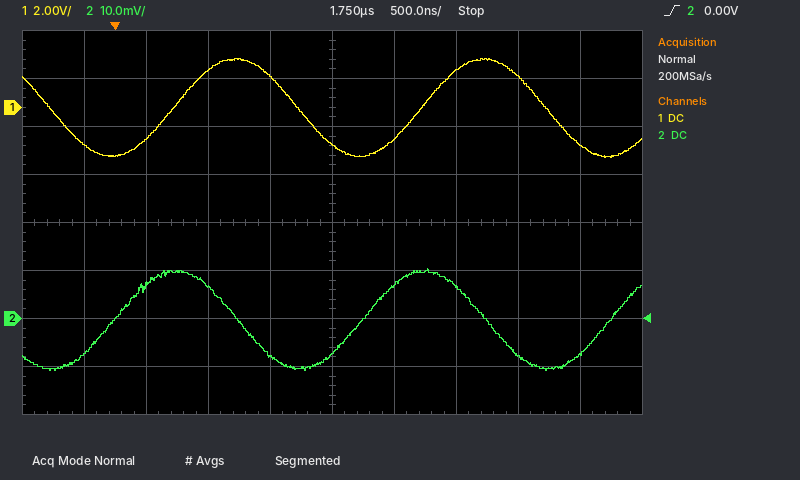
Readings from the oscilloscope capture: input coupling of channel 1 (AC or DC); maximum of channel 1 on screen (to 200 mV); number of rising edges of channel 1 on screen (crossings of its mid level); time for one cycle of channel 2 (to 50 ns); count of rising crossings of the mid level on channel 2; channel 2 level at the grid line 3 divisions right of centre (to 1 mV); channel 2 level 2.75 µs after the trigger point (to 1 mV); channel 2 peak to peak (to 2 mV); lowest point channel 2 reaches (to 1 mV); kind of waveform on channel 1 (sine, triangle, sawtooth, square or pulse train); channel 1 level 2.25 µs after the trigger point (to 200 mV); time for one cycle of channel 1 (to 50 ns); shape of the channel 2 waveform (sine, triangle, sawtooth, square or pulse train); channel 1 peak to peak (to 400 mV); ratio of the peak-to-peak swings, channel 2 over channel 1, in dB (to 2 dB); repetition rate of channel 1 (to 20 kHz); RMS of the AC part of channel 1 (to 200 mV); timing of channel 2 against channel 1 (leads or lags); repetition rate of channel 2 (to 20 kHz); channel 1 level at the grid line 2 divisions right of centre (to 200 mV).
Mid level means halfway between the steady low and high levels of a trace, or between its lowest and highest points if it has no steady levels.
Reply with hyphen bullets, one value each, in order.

- DC
- 2.0 V
- 2
- 2.00 µs
- 3
- -8 mV
- 7 mV
- 22 mV
- -11 mV
- sine
- -1.4 V
- 2.00 µs
- sine
- 4.0 V
- -46 dB
- 500 kHz
- 1.4 V
- leads
- 500 kHz
- 1.6 V
